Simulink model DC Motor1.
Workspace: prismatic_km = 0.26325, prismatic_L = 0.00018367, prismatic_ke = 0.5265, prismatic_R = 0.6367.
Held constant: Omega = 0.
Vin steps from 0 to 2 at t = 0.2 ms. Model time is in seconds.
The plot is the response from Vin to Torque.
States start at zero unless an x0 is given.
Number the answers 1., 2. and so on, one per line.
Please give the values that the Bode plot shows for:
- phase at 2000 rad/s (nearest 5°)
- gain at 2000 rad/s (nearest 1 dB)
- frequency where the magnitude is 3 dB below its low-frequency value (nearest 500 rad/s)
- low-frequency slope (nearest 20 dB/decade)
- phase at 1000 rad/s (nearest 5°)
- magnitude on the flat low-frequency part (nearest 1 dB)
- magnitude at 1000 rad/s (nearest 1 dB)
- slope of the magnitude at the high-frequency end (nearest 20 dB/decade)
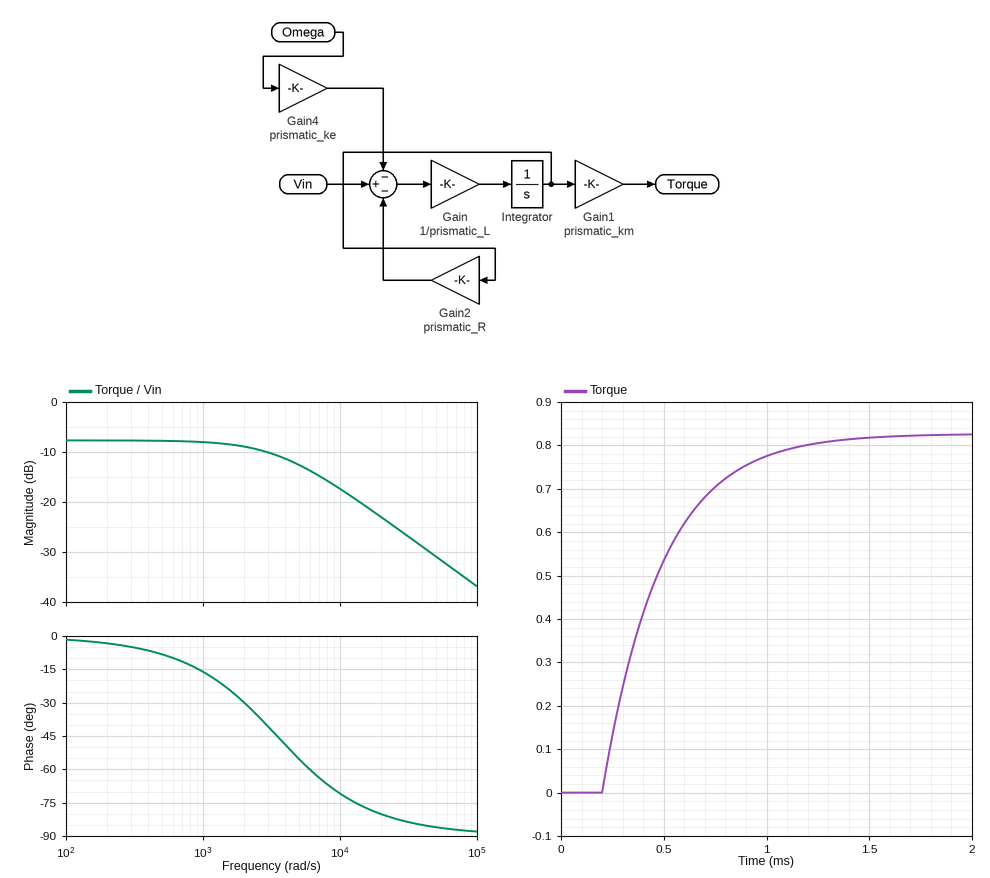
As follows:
1. -30°
2. -9 dB
3. 3500 rad/s
4. 0 dB/decade
5. -15°
6. -8 dB
7. -8 dB
8. -20 dB/decade
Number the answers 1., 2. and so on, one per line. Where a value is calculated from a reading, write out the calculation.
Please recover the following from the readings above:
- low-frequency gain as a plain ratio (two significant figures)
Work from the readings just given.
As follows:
1. 10^(-8 / 20) = 0.40
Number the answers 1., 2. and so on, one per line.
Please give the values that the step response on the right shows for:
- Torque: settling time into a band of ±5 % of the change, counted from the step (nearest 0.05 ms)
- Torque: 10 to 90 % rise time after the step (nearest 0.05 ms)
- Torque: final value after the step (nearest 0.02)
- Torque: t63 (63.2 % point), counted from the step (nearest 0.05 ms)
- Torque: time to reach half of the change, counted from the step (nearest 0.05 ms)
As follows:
1. 0.85 ms
2. 0.65 ms
3. 0.82
4. 0.30 ms
5. 0.20 ms
